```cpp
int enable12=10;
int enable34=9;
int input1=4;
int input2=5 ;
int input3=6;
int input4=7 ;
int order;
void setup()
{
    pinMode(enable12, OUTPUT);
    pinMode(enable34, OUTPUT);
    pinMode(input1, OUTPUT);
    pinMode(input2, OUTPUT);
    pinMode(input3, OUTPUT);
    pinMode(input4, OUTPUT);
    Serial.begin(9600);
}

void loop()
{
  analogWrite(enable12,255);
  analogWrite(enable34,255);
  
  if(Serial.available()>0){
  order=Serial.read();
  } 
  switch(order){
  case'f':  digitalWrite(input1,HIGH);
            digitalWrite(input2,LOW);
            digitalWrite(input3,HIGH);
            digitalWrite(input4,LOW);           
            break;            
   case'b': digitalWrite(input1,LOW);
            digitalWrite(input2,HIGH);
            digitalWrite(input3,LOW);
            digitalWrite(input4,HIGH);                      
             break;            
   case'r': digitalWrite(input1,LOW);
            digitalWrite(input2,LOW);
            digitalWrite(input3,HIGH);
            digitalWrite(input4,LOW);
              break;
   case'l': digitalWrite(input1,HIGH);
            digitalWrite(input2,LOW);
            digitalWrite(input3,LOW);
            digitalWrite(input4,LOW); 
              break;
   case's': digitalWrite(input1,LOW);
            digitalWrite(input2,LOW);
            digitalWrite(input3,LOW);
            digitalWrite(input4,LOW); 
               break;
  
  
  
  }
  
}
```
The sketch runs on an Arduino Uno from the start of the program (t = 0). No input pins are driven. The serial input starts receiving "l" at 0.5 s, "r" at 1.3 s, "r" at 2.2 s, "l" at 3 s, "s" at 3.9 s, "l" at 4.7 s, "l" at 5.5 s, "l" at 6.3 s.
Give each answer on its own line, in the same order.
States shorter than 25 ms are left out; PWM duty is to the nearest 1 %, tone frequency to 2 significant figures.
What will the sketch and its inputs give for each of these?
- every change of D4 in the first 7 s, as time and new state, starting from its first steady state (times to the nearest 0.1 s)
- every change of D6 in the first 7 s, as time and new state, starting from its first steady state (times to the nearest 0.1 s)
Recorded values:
0 s low; 0.5 s high; 1.3 s low; 3 s high; 3.9 s low; 4.7 s high
0 s low; 1.3 s high; 3 s low
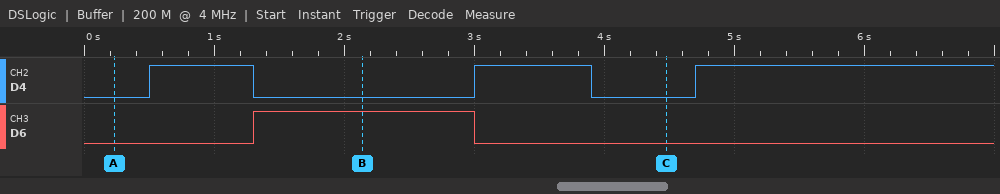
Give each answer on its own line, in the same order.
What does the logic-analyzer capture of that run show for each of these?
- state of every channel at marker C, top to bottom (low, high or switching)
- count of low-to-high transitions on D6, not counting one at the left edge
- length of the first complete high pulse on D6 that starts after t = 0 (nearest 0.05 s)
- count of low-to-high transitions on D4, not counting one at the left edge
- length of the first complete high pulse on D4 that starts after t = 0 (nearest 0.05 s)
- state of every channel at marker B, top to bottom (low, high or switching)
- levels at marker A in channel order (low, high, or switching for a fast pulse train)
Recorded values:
D4 low, D6 low
1
1.70 s
3
0.80 s
D4 low, D6 high
D4 low, D6 low
